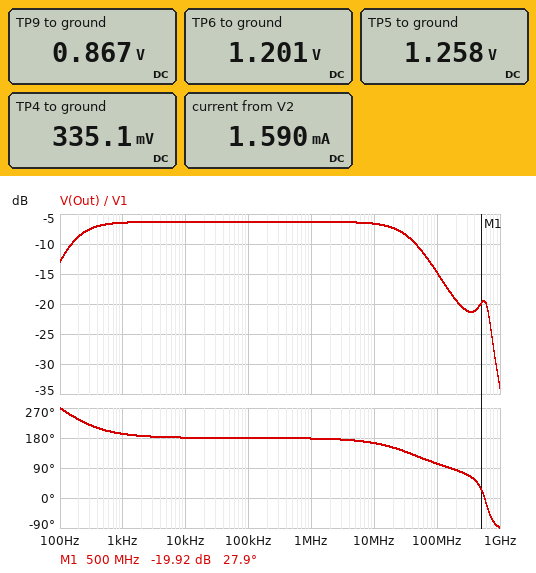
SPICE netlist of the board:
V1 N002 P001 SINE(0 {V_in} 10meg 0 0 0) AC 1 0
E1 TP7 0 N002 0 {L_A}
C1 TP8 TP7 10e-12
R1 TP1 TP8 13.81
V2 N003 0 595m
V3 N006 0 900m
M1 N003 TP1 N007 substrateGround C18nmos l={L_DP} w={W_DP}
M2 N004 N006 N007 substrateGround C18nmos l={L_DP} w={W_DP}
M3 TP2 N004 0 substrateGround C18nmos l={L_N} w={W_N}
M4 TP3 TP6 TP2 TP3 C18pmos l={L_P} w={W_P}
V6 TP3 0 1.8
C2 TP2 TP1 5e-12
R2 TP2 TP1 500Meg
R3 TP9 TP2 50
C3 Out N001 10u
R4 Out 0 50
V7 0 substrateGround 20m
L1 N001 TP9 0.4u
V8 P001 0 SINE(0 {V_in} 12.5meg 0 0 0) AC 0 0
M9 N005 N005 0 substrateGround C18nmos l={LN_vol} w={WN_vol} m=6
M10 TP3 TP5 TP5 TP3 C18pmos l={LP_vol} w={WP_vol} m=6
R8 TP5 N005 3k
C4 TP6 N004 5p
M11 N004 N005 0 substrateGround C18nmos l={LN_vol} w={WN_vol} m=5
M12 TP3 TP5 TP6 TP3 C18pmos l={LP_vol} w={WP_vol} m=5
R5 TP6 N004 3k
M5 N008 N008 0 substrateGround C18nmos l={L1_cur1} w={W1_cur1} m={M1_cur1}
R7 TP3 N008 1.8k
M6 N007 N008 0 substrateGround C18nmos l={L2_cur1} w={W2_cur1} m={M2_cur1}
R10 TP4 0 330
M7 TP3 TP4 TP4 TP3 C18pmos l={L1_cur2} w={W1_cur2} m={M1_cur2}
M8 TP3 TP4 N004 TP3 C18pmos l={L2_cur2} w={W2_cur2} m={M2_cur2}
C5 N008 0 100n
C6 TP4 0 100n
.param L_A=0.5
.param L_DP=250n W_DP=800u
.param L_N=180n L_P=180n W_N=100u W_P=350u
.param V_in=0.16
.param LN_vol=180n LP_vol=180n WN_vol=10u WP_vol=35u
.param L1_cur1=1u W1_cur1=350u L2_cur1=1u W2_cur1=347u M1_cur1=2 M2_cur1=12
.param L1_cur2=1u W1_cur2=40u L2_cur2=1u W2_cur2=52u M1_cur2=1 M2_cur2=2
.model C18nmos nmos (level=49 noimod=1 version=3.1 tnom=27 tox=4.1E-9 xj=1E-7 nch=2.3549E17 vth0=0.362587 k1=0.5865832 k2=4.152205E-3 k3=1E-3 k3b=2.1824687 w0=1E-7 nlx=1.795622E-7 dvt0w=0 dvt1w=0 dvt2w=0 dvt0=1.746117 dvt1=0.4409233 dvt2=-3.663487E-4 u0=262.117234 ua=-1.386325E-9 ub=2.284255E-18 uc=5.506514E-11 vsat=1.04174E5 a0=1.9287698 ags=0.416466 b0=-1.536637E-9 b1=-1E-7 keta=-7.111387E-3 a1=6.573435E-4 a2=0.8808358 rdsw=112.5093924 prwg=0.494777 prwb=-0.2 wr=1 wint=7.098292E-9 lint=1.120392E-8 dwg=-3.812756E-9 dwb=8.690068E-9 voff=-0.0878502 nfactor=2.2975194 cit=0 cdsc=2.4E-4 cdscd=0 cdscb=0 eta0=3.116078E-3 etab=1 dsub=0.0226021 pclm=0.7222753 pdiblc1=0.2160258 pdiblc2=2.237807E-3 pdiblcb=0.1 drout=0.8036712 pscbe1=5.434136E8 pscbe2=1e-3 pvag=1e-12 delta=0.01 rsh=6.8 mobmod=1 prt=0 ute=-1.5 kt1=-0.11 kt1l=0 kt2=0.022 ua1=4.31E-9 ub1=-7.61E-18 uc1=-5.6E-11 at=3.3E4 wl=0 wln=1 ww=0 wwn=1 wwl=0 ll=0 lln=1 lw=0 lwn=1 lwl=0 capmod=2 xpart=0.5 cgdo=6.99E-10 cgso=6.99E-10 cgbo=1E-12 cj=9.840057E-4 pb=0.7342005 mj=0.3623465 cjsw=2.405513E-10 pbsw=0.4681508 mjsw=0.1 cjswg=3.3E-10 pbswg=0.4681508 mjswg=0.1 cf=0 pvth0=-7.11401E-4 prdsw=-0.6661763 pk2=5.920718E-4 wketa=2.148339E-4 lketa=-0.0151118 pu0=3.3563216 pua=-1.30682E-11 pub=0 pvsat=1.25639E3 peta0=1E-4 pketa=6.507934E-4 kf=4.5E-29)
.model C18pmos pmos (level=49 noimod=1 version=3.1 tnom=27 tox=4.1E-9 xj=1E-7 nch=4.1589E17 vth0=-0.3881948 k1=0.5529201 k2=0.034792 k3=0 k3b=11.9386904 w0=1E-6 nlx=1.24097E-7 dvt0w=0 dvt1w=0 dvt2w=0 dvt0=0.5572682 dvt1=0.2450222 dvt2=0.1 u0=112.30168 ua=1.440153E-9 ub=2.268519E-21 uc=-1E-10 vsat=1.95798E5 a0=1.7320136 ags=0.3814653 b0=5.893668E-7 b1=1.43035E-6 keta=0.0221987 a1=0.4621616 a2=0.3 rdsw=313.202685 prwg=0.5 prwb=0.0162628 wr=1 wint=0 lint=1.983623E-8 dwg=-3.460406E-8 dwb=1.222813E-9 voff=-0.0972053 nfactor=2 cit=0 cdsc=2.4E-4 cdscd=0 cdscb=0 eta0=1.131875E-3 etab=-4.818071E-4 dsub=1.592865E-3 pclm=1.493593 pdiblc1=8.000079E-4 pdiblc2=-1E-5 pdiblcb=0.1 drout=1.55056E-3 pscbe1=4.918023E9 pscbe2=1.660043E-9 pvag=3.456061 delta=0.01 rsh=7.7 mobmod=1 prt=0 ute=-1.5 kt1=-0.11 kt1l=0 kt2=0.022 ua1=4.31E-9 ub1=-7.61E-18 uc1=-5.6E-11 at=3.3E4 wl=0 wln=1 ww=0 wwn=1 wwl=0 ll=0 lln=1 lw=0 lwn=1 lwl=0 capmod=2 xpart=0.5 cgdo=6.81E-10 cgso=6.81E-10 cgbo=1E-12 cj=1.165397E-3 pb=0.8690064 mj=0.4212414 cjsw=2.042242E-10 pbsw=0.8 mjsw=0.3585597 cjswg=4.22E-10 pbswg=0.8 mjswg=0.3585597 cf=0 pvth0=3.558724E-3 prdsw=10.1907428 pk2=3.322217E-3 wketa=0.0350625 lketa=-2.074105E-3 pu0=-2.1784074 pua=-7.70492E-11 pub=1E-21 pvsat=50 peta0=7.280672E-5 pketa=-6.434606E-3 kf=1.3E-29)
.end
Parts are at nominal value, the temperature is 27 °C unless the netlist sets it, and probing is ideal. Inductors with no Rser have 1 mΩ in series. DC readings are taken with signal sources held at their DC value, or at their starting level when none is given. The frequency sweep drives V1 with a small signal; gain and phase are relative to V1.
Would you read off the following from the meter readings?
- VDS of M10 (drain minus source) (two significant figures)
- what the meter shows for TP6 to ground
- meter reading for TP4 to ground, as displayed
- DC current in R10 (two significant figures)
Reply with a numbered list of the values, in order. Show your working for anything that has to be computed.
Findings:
1. 1.8 V - 1.258 V = 540 mV
2. 1.201 V
3. 335.1 mV
4. (335.1 mV) / 330 Ω = 1.0 mA
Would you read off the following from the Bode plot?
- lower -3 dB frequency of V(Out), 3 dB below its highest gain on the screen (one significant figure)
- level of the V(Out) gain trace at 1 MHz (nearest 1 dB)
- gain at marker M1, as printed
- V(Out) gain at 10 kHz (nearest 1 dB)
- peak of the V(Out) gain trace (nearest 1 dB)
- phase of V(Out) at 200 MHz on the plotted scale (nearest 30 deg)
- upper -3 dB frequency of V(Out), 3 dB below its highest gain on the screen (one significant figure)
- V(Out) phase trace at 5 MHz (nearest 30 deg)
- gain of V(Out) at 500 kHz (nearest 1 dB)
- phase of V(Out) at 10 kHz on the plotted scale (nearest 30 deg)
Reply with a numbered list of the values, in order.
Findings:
1. 200 Hz
2. -6 dB
3. -19.92 dB
4. -6 dB
5. -6 dB
6. 90 deg
7. 40 MHz
8. 180 deg
9. -6 dB
10. 180 deg
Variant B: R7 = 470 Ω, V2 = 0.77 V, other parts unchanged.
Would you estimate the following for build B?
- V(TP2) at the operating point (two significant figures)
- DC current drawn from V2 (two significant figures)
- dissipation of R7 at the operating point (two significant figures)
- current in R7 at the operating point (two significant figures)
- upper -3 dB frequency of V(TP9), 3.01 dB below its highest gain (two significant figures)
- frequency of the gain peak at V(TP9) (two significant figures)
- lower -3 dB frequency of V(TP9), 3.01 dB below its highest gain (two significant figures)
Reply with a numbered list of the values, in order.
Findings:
1. 1.1 V
2. 12 mA
3. 3.0 mW
4. 2.5 mA
5. 940 MHz
6. 750 MHz
7. 570 MHz
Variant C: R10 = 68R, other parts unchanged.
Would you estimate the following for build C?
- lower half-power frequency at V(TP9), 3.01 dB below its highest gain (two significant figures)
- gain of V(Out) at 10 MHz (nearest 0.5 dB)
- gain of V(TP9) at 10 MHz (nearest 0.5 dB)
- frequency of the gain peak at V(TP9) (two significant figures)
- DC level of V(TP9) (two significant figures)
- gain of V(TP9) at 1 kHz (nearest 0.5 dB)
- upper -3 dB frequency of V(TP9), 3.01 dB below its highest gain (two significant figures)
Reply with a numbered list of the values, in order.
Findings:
1. 290 MHz
2. -7.0 dB
3. -6.0 dB
4. 420 MHz
5. 770 mV
6. -6.5 dB
7. 560 MHz
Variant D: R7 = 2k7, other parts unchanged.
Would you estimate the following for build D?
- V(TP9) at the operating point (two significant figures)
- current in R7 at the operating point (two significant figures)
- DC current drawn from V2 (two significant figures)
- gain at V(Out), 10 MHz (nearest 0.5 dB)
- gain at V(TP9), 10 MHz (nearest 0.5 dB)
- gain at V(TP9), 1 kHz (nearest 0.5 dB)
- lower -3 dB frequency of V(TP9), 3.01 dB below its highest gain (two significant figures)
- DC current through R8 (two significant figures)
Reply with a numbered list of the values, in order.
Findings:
1. 770 mV
2. 480 µA
3. 240 µA
4. -7.0 dB
5. -6.0 dB
6. -6.5 dB
7. 210 MHz
8. 240 µA
